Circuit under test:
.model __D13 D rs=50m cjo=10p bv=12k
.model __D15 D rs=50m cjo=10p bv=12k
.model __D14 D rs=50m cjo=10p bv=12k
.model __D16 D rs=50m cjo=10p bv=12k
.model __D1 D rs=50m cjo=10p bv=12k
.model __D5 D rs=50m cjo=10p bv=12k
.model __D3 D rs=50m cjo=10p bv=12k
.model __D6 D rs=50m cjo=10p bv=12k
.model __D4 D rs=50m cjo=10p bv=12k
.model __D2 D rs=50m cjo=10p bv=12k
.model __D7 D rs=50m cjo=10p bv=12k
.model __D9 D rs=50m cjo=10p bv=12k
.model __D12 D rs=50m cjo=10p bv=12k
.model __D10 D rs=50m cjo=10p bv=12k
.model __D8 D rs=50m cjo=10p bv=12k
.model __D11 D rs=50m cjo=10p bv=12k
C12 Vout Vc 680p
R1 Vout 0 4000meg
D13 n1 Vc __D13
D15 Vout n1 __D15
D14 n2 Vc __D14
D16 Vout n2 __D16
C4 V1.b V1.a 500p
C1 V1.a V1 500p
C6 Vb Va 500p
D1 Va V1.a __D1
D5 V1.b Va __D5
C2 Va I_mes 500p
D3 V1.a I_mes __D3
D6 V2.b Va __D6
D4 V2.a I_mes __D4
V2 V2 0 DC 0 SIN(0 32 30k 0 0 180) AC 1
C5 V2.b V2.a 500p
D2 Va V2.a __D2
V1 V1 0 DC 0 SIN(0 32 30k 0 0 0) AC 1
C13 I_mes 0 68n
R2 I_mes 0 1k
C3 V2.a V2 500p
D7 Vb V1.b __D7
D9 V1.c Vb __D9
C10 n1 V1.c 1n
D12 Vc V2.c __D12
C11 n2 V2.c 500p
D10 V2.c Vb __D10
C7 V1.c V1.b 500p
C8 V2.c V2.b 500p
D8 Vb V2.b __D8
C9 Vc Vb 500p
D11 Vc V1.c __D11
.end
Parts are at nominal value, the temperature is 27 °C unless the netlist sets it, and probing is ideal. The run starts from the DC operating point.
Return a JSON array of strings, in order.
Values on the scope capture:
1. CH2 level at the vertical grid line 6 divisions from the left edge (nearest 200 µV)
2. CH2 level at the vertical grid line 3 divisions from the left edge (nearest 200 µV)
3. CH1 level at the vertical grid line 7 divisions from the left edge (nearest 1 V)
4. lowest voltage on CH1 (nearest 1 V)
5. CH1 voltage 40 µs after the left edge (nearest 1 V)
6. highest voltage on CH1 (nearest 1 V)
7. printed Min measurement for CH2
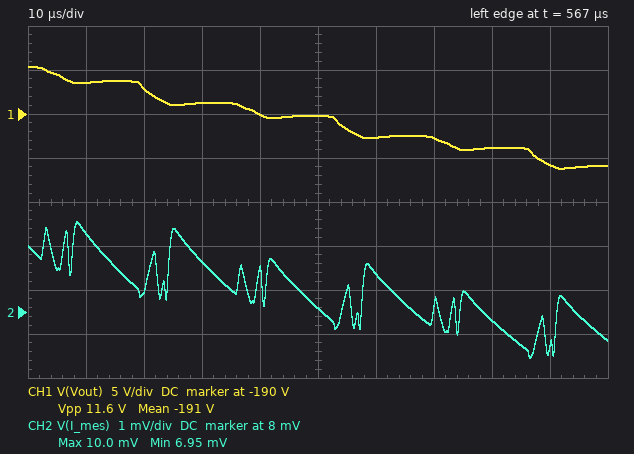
["8.8 mV", "9.2 mV", "-193 V", "-196 V", "-190 V", "-185 V", "6.95 mV"]
